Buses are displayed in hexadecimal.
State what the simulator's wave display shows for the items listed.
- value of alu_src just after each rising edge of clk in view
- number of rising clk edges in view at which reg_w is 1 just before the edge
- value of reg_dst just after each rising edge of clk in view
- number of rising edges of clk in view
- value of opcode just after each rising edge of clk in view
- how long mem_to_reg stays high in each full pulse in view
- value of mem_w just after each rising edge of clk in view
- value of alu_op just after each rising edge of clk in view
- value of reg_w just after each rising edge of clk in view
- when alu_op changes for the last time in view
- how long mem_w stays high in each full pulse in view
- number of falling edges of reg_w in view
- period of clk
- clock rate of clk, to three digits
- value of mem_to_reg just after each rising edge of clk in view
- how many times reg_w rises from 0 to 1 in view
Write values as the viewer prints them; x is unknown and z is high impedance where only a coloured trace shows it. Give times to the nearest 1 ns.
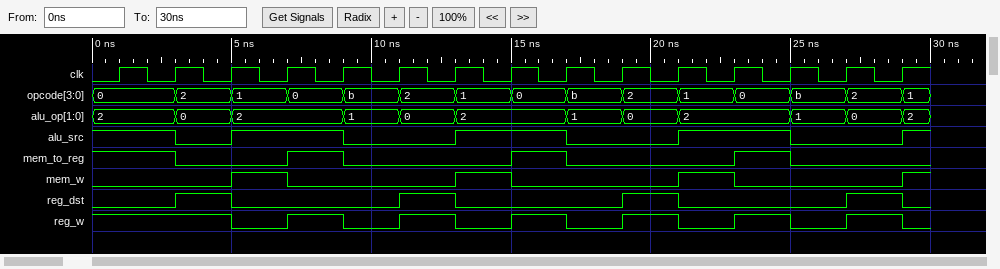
1 0 1 1 0 0 1 1 0 0 1 1 0 0 1
9
0 1 0 0 0 1 0 0 0 1 0 0 0 1 0
15
0, 2, 1, 0, b, 2, 1, 0, b, 2, 1, 0, b, 2, 1
2 ns, 2 ns, 2 ns
0 0 1 0 0 0 1 0 0 0 1 0 0 0 1
2, 0, 2, 2, 1, 0, 2, 2, 1, 0, 2, 2, 1, 0, 2
1 1 0 1 0 1 0 1 0 1 0 1 0 1 0
29 ns
2 ns, 2 ns, 2 ns
7
2 ns
500 MHz
1 0 0 1 0 0 0 1 0 0 0 1 0 0 0
6
